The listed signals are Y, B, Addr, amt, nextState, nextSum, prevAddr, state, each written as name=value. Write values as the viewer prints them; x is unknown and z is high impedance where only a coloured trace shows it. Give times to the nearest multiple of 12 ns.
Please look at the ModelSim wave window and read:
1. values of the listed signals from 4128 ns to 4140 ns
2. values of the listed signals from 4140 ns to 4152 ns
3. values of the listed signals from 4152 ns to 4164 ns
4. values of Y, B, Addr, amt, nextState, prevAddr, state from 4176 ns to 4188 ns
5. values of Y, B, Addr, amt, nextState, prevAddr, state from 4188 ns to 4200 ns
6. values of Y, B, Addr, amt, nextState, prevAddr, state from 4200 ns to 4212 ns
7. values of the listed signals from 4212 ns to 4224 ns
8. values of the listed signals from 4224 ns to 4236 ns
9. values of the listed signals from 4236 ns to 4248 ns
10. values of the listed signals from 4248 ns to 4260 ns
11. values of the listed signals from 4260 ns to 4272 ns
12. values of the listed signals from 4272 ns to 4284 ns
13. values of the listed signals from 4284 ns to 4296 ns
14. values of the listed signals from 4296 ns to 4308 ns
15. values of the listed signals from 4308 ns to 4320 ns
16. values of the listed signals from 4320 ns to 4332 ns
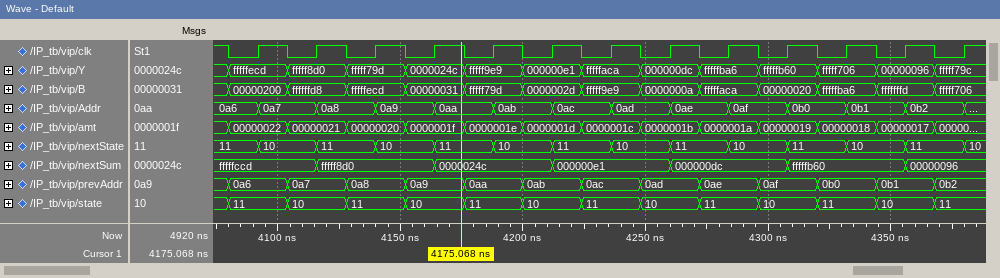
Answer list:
Y=fffff79d, B=fffffecd, Addr=0a8, amt=00000020, nextState=11, nextSum=fffff8d0, prevAddr=0a8, state=11
Y=fffff79d, B=fffffecd, Addr=0a9, amt=00000020, nextState=10, nextSum=fffff8d0, prevAddr=0a8, state=11
Y=0000024c, B=00000031, Addr=0a9, amt=0000001f, nextState=10, nextSum=fffff8d0, prevAddr=0a9, state=10
Y=fffff9e9, B=fffff79d, Addr=0aa, amt=0000001e, nextState=11, prevAddr=0aa, state=11
Y=fffff9e9, B=fffff79d, Addr=0ab, amt=0000001e, nextState=10, prevAddr=0aa, state=11
Y=000000e1, B=0000002d, Addr=0ab, amt=0000001d, nextState=10, prevAddr=0ab, state=10
Y=000000e1, B=0000002d, Addr=0ac, amt=0000001d, nextState=11, nextSum=000000e1, prevAddr=0ab, state=10
Y=fffffaca, B=fffff9e9, Addr=0ac, amt=0000001c, nextState=11, nextSum=000000e1, prevAddr=0ac, state=11
Y=fffffaca, B=fffff9e9, Addr=0ad, amt=0000001c, nextState=10, nextSum=000000e1, prevAddr=0ac, state=11
Y=000000dc, B=0000000a, Addr=0ad, amt=0000001b, nextState=10, nextSum=000000e1, prevAddr=0ad, state=10
Y=000000dc, B=0000000a, Addr=0ae, amt=0000001b, nextState=11, nextSum=000000dc, prevAddr=0ad, state=10
Y=fffffba6, B=fffffaca, Addr=0ae, amt=0000001a, nextState=11, nextSum=000000dc, prevAddr=0ae, state=11
Y=fffffba6, B=fffffaca, Addr=0af, amt=0000001a, nextState=10, nextSum=000000dc, prevAddr=0ae, state=11
Y=fffffb60, B=00000020, Addr=0af, amt=00000019, nextState=10, nextSum=000000dc, prevAddr=0af, state=10
Y=fffffb60, B=00000020, Addr=0b0, amt=00000019, nextState=11, nextSum=fffffb60, prevAddr=0af, state=10
Y=fffff706, B=fffffba6, Addr=0b0, amt=00000018, nextState=11, nextSum=fffffb60, prevAddr=0b0, state=11
